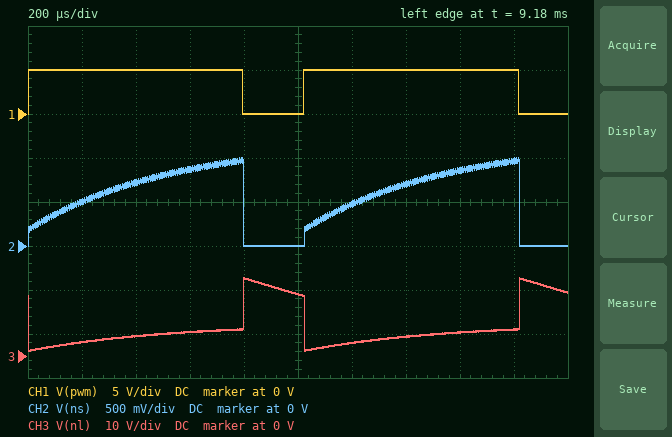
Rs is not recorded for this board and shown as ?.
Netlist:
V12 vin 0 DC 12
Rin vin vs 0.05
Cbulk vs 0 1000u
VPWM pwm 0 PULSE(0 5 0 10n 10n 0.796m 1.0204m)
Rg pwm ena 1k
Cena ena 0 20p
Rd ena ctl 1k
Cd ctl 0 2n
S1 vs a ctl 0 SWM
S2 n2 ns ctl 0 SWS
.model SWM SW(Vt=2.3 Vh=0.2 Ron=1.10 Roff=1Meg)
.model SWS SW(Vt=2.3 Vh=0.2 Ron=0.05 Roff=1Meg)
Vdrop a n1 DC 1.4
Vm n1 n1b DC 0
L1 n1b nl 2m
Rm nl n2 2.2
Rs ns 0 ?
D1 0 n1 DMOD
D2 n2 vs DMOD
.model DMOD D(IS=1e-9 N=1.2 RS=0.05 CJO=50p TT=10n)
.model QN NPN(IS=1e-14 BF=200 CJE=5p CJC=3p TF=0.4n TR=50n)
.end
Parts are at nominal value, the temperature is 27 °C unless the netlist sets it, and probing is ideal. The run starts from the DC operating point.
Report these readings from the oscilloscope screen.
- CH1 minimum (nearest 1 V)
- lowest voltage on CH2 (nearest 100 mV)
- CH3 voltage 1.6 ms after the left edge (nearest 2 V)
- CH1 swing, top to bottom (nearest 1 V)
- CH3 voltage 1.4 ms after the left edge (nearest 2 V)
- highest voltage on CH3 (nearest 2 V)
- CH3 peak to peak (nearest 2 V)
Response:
0 V
0 V
6 V
5 V
4 V
18 V
16 V
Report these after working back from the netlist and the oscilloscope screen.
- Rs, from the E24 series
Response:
0.43 Ω
